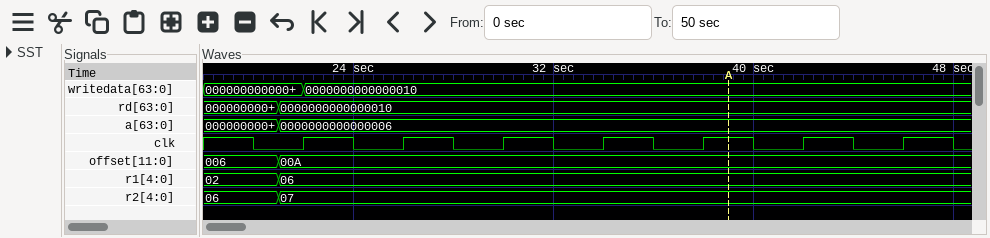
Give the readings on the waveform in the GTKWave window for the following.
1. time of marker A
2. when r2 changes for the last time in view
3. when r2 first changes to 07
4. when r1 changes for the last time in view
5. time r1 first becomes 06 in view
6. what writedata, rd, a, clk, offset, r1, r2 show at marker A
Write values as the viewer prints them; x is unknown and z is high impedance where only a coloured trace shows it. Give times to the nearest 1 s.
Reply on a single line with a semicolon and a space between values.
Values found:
39 s; 21 s; 21 s; 21 s; 21 s; writedata=0000000000000010, rd=0000000000000010, a=0000000000000006, clk=1, offset=00A, r1=06, r2=07
